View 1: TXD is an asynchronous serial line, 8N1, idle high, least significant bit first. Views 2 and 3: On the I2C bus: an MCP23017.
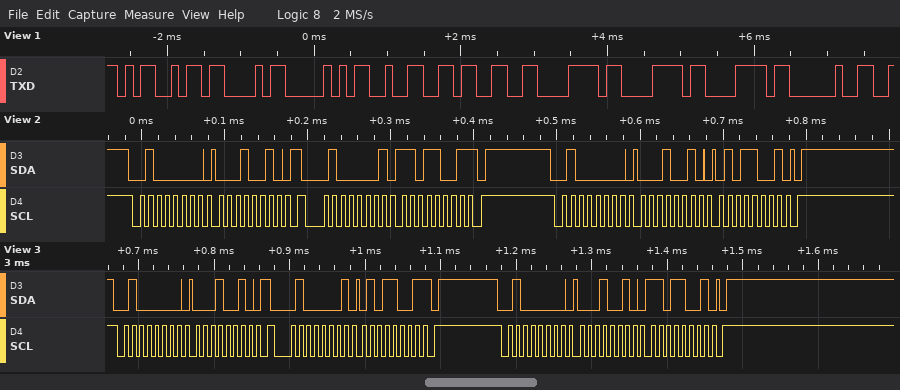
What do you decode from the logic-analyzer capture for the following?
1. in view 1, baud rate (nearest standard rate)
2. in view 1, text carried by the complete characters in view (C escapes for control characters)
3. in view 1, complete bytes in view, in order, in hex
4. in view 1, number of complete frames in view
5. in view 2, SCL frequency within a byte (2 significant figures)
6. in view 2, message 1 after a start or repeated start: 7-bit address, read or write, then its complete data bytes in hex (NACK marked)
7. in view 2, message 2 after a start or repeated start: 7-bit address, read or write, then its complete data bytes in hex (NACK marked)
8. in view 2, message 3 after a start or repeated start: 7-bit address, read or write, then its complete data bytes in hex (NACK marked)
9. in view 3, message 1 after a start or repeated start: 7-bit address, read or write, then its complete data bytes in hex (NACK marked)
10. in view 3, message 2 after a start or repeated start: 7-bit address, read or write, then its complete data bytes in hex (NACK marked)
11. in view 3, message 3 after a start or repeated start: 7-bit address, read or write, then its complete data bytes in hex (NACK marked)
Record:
9600 baud
"MCP23xxx "
4D 43 50 32 33 78 78 78 20
9
100 kHz
0x20 write: 12
0x20 read: D9 NACK
0x20 write: 12 59
0x20 write: 12
0x20 read: 59 NACK
0x20 write: 12 D9
